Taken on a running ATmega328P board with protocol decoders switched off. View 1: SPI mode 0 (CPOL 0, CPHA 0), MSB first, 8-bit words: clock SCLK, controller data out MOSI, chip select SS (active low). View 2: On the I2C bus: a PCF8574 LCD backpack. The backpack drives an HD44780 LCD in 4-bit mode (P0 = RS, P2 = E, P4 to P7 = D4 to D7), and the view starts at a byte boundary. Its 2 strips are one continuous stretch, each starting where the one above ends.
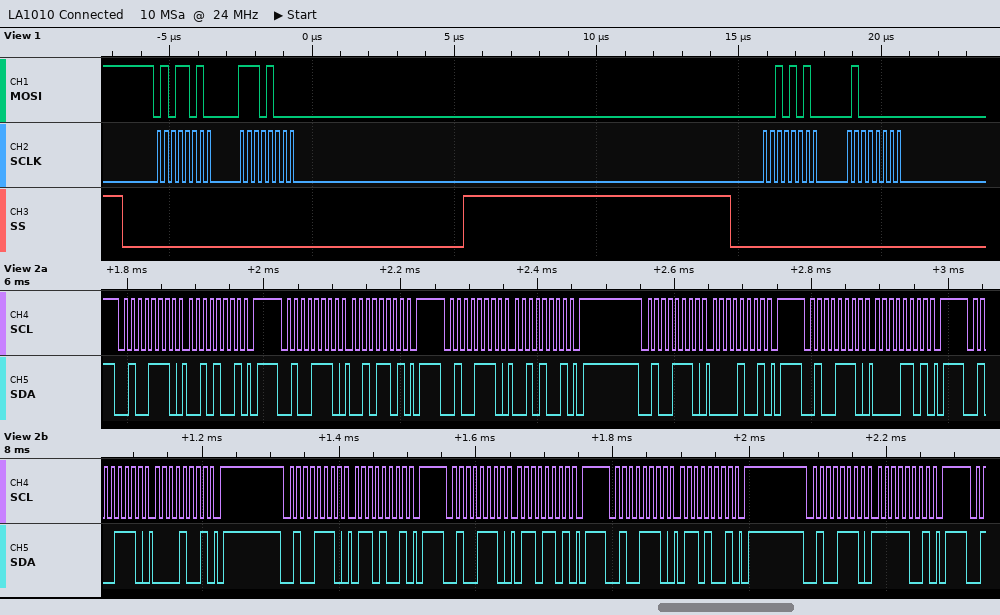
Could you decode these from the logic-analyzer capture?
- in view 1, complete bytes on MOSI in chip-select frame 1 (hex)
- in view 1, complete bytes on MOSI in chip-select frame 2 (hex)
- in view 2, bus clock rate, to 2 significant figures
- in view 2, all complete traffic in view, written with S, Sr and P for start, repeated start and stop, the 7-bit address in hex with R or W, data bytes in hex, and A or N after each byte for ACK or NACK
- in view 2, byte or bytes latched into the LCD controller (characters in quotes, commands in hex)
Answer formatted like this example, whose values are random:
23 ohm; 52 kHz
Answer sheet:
5A E8; 2A 40; 100 kHz; S 27W A 29 A P S 27W A 2D A P S 27W A 29 A P S 27W A 09 A P S 27W A 0D A P S 27W A 09 A P S 27W A 69 A P S 27W A 6D A P S 27W A 69 A P S 27W A F9 A P; ' '
